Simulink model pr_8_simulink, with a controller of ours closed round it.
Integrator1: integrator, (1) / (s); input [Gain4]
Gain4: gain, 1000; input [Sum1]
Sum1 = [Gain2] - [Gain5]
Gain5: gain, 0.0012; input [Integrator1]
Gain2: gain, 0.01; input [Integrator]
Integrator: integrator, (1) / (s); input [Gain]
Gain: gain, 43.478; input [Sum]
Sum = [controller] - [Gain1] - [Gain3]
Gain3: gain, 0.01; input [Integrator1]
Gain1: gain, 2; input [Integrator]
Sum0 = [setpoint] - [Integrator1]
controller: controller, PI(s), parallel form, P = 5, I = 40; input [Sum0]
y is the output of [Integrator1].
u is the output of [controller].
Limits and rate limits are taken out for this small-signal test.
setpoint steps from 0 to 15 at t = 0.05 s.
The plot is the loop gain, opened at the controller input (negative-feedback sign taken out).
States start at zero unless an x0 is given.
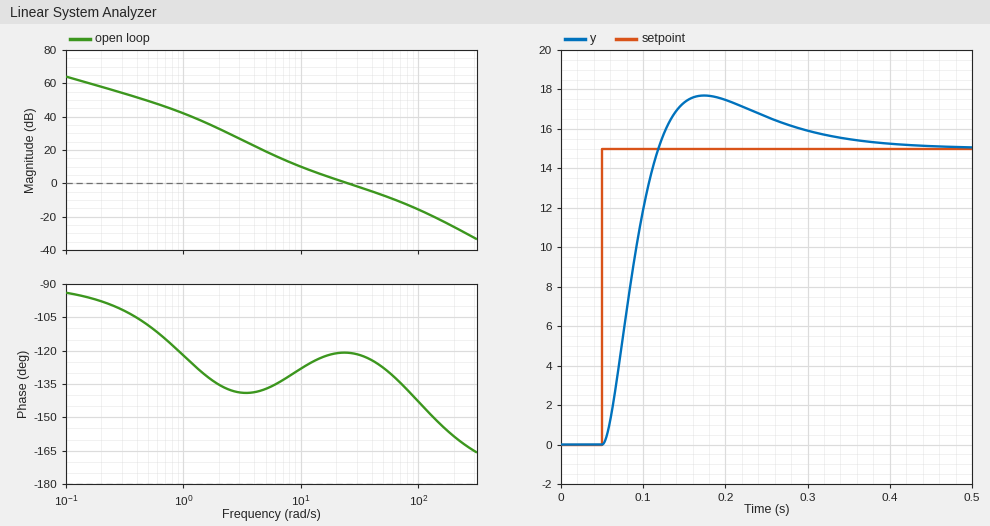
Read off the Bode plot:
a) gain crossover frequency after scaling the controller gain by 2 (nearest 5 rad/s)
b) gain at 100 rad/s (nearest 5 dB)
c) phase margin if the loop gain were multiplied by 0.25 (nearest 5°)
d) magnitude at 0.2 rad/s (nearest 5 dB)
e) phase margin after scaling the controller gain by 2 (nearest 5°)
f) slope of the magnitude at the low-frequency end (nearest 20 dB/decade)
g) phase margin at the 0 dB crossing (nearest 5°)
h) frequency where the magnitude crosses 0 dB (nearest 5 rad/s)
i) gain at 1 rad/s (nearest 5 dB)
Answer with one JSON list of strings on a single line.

["45 rad/s", "-15 dB", "50°", "60 dB", "55°", "-20 dB/decade", "60°", "25 rad/s", "40 dB"]
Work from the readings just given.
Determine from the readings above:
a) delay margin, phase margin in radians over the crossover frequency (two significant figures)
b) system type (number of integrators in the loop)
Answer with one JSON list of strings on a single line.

["0.042 s", "1"]
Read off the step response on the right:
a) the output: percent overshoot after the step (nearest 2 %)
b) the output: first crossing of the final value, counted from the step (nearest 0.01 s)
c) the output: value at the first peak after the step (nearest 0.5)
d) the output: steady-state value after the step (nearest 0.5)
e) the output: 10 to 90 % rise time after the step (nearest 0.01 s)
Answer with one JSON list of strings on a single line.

["18 %", "0.07 s", "17.5", "15.0", "0.05 s"]
